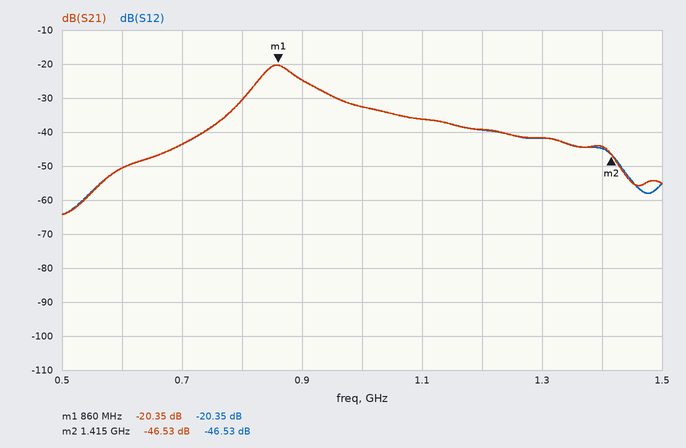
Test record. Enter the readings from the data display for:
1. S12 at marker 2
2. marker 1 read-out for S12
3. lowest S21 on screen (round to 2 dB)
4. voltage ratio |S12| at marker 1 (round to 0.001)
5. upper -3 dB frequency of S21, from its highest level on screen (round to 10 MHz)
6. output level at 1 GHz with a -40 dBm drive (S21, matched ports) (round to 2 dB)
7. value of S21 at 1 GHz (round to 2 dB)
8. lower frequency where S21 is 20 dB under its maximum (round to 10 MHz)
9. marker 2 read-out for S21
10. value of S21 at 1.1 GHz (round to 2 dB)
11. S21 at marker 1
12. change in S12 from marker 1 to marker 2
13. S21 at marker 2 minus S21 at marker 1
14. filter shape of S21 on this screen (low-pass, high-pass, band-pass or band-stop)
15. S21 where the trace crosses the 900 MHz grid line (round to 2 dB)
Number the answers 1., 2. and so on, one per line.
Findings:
1. -46.53 dB
2. -20.35 dB
3. -64 dB
4. 0.096
5. 890 MHz
6. -72 dBm
7. -32 dB
8. 730 MHz
9. -46.53 dB
10. -36 dB
11. -20.35 dB
12. -26.18 dB
13. -26.18 dB
14. band-pass
15. -24 dB
